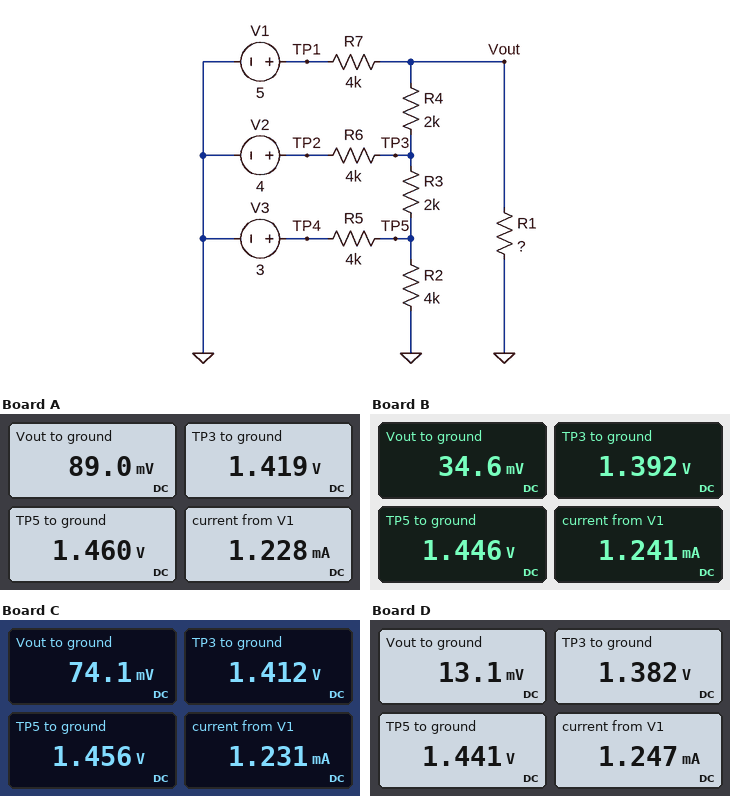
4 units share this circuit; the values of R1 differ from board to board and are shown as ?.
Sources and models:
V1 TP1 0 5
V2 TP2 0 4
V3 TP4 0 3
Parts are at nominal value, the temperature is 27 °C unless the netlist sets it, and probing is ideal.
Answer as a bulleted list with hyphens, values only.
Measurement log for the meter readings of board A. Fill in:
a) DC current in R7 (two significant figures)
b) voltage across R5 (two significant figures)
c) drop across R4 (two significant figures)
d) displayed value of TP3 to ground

- 1.2 mA
- 1.5 V
- 1.3 V
- 1.419 V
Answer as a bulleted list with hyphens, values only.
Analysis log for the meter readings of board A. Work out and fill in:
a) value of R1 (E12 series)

- 47 Ω
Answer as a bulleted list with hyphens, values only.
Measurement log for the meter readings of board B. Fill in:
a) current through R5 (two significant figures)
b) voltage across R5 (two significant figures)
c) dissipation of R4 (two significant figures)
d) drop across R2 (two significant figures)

- 390 µA
- 1.6 V
- 920 µW
- 1.4 V
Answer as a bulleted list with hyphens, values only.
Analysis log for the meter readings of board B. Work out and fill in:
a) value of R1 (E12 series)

- 18 Ω
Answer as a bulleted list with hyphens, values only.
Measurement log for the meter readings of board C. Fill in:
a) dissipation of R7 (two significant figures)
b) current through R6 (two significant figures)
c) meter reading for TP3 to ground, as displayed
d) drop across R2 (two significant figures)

- 6.1 mW
- 650 µA
- 1.412 V
- 1.5 V
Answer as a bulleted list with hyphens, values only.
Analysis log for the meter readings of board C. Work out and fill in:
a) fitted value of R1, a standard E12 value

- 39 Ω
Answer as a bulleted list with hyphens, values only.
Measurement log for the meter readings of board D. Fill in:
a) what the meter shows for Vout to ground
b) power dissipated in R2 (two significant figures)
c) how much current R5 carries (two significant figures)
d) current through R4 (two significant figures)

- 13.1 mV
- 520 µW
- 390 µA
- 680 µA
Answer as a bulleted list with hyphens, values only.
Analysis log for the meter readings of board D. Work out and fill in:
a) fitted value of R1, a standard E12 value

- 6.8 Ω
